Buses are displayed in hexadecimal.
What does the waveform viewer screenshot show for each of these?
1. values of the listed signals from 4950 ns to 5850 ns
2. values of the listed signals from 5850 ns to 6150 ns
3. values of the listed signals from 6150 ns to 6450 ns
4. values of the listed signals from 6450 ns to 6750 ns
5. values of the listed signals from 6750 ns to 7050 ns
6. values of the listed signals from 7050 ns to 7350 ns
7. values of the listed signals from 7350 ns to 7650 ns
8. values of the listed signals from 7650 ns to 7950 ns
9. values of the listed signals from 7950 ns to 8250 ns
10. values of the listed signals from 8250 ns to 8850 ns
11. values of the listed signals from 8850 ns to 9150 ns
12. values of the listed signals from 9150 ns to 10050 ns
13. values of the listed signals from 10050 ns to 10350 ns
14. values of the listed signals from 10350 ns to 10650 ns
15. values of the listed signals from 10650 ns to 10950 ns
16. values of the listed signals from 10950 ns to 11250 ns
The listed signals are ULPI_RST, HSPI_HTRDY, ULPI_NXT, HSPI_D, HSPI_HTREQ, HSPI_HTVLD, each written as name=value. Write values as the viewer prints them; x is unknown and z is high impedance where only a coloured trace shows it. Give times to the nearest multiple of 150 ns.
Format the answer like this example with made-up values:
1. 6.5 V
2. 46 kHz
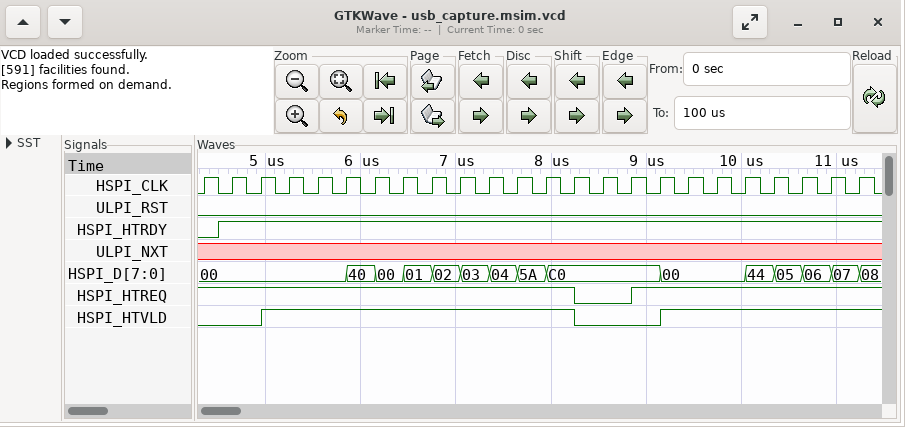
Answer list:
1. ULPI_RST=0, HSPI_HTRDY=1, ULPI_NXT=x, HSPI_D=00, HSPI_HTREQ=1, HSPI_HTVLD=1
2. ULPI_RST=0, HSPI_HTRDY=1, ULPI_NXT=x, HSPI_D=40, HSPI_HTREQ=1, HSPI_HTVLD=1
3. ULPI_RST=0, HSPI_HTRDY=1, ULPI_NXT=x, HSPI_D=00, HSPI_HTREQ=1, HSPI_HTVLD=1
4. ULPI_RST=0, HSPI_HTRDY=1, ULPI_NXT=x, HSPI_D=01, HSPI_HTREQ=1, HSPI_HTVLD=1
5. ULPI_RST=0, HSPI_HTRDY=1, ULPI_NXT=x, HSPI_D=02, HSPI_HTREQ=1, HSPI_HTVLD=1
6. ULPI_RST=0, HSPI_HTRDY=1, ULPI_NXT=x, HSPI_D=03, HSPI_HTREQ=1, HSPI_HTVLD=1
7. ULPI_RST=0, HSPI_HTRDY=1, ULPI_NXT=x, HSPI_D=04, HSPI_HTREQ=1, HSPI_HTVLD=1
8. ULPI_RST=0, HSPI_HTRDY=1, ULPI_NXT=x, HSPI_D=5A, HSPI_HTREQ=1, HSPI_HTVLD=1
9. ULPI_RST=0, HSPI_HTRDY=1, ULPI_NXT=x, HSPI_D=C0, HSPI_HTREQ=1, HSPI_HTVLD=1
10. ULPI_RST=0, HSPI_HTRDY=1, ULPI_NXT=x, HSPI_D=C0, HSPI_HTREQ=0, HSPI_HTVLD=0
11. ULPI_RST=0, HSPI_HTRDY=1, ULPI_NXT=x, HSPI_D=C0, HSPI_HTREQ=1, HSPI_HTVLD=0
12. ULPI_RST=0, HSPI_HTRDY=1, ULPI_NXT=x, HSPI_D=00, HSPI_HTREQ=1, HSPI_HTVLD=1
13. ULPI_RST=0, HSPI_HTRDY=1, ULPI_NXT=x, HSPI_D=44, HSPI_HTREQ=1, HSPI_HTVLD=1
14. ULPI_RST=0, HSPI_HTRDY=1, ULPI_NXT=x, HSPI_D=05, HSPI_HTREQ=1, HSPI_HTVLD=1
15. ULPI_RST=0, HSPI_HTRDY=1, ULPI_NXT=x, HSPI_D=06, HSPI_HTREQ=1, HSPI_HTVLD=1
16. ULPI_RST=0, HSPI_HTRDY=1, ULPI_NXT=x, HSPI_D=07, HSPI_HTREQ=1, HSPI_HTVLD=1
